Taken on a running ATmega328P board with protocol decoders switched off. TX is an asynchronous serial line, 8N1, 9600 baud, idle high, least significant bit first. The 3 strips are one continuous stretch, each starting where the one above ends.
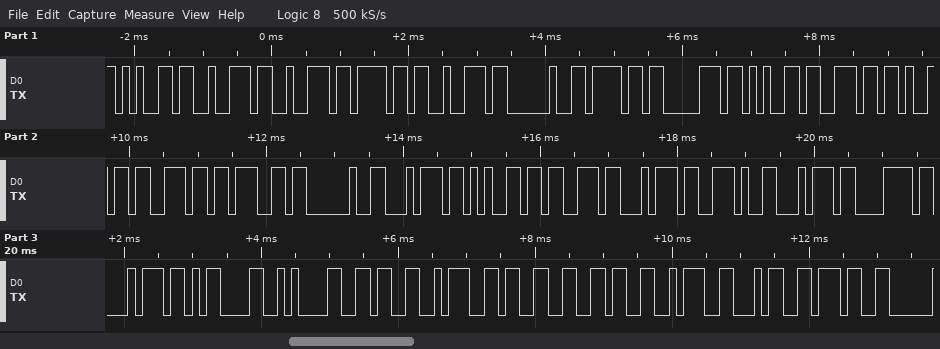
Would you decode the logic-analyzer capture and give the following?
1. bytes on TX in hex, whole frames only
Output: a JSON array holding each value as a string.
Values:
["65 72 72 6F 72 20 6F 70 65 6E 69 6E 67 20 74 65 73 74 2E 74 78 74 0D 0A 36 3A 33 36 3A 34 37"]
